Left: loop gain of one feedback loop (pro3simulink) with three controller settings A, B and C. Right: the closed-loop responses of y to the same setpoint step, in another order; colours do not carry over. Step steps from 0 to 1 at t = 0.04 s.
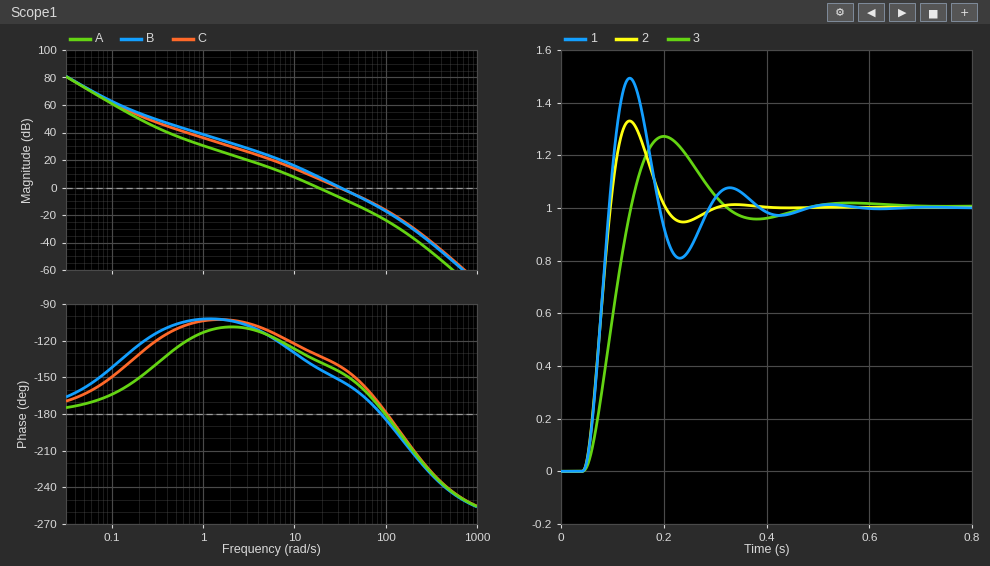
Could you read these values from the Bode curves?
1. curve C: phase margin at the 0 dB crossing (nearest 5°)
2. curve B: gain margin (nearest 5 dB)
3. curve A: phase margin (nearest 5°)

40°
15 dB
45°
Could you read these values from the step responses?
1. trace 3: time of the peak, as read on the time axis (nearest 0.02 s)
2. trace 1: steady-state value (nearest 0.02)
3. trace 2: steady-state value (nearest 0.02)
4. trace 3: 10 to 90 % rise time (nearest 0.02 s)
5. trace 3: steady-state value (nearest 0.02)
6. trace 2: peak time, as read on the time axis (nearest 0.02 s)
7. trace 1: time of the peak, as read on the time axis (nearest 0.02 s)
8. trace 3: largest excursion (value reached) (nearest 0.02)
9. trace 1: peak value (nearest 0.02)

0.20 s
1.00
1.00
0.06 s
1.00
0.14 s
0.14 s
1.28
1.50
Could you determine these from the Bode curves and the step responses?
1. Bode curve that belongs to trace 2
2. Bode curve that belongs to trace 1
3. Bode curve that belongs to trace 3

C
B
A
